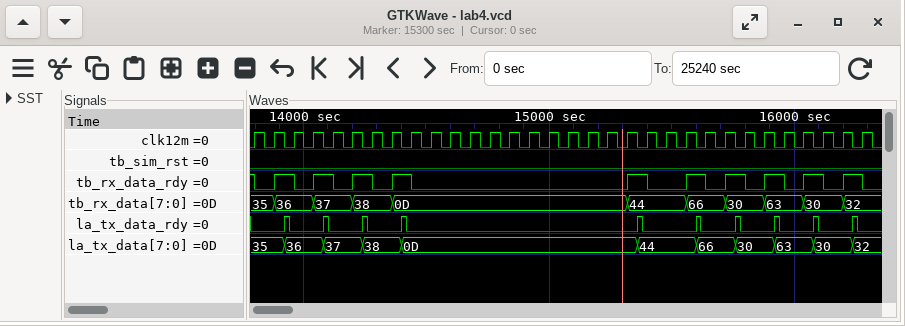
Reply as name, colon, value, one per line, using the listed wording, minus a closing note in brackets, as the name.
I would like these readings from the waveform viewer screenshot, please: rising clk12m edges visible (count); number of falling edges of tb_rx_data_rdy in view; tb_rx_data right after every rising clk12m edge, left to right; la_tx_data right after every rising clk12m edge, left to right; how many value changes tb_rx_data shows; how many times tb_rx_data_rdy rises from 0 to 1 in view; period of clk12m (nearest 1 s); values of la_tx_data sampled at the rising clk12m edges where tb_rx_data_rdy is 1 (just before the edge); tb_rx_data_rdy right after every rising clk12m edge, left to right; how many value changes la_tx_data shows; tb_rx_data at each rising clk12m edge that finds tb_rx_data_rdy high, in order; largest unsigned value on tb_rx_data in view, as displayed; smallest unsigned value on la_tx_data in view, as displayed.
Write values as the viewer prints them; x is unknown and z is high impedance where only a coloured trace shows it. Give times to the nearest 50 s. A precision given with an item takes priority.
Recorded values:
rising clk12m edges visible: 32
number of falling edges of tb_rx_data_rdy in view: 11
tb_rx_data right after every rising clk12m edge, left to right: 35, 36, 36, 37, 37, 38, 38, 0D, 0D, 0D, 0D, 0D, 0D, 0D, 0D, 0D, 0D, 0D, 0D, 44, 44, 44, 66, 66, 30, 30, 63, 63, 30, 30, 32, 32
la_tx_data right after every rising clk12m edge, left to right: 35, 35, 36, 36, 37, 37, 38, 38, 0D, 0D, 0D, 0D, 0D, 0D, 0D, 0D, 0D, 0D, 0D, 0D, 44, 44, 44, 66, 66, 30, 30, 63, 63, 30, 30, 32
how many value changes tb_rx_data shows: 10
how many times tb_rx_data_rdy rises from 0 to 1 in view: 10
period of clk12m: 80 s
values of la_tx_data sampled at the rising clk12m edges where tb_rx_data_rdy is 1: 35, 36, 37, 38, 0D, 44, 66, 30, 63, 30, 32
tb_rx_data_rdy right after every rising clk12m edge, left to right: 0 1 0 1 0 1 0 1 0 0 0 0 0 0 0 0 0 0 0 1 0 0 1 0 1 0 1 0 1 0 1 0
how many value changes la_tx_data shows: 10
tb_rx_data at each rising clk12m edge that finds tb_rx_data_rdy high, in order: 35, 36, 37, 38, 0D, 44, 66, 30, 63, 30, 32
largest unsigned value on tb_rx_data in view, as displayed: 66
smallest unsigned value on la_tx_data in view, as displayed: 0D
